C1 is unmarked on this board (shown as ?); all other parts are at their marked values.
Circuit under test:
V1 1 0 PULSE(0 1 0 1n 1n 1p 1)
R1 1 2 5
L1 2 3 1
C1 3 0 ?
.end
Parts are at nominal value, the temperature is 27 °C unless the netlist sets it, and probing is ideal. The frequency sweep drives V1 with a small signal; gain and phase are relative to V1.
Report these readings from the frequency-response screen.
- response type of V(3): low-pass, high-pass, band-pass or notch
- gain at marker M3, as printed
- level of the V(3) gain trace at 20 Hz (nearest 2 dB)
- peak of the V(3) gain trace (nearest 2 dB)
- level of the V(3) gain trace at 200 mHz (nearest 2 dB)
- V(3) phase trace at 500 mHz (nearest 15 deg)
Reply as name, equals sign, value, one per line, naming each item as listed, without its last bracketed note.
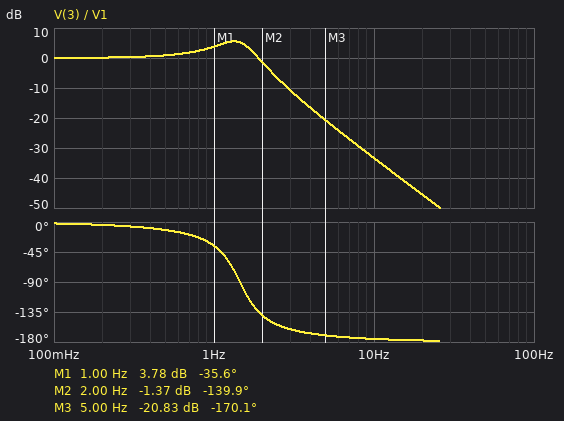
response type of V(3): low-pass, high-pass, band-pass or notch = low-pass
gain at marker M3, as printed = -20.83 dB
level of the V(3) gain trace at 20 Hz = -46 dB
peak of the V(3) gain trace = 6 dB
level of the V(3) gain trace at 200 mHz = 0 dB
V(3) phase trace at 500 mHz = -15 deg
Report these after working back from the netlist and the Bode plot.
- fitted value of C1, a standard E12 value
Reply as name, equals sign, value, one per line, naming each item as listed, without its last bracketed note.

fitted value of C1, a standard E12 value = 12 mF
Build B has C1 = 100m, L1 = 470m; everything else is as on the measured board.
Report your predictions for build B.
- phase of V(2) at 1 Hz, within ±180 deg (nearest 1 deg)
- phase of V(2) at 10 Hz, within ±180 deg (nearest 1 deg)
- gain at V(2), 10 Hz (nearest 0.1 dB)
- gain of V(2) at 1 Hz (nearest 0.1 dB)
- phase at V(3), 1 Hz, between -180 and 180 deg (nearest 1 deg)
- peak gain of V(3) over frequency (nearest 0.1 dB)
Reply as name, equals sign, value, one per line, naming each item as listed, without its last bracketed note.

phase of V(2) at 1 Hz, within ±180 deg = 75 deg
phase of V(2) at 10 Hz, within ±180 deg = 10 deg
gain at V(2), 10 Hz = -0.1 dB
gain of V(2) at 1 Hz = -11.6 dB
phase at V(3), 1 Hz, between -180 and 180 deg = -105 deg
peak gain of V(3) over frequency = 0 dB
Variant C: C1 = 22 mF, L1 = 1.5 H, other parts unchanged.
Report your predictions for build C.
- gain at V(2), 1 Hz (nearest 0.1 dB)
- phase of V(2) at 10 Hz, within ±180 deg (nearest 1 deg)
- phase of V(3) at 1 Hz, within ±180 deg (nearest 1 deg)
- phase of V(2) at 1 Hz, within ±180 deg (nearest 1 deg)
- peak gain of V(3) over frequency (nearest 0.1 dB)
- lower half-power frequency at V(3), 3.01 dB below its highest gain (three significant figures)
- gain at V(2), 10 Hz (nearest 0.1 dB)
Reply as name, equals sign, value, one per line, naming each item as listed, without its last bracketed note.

gain at V(2), 1 Hz = -7.9 dB
phase of V(2) at 10 Hz, within ±180 deg = 3 deg
phase of V(3) at 1 Hz, within ±180 deg = -114 deg
phase of V(2) at 1 Hz, within ±180 deg = 66 deg
peak gain of V(3) over frequency = 4.8 dB
lower half-power frequency at V(3), 3.01 dB below its highest gain = 429 mHz
gain at V(2), 10 Hz = 0 dB
